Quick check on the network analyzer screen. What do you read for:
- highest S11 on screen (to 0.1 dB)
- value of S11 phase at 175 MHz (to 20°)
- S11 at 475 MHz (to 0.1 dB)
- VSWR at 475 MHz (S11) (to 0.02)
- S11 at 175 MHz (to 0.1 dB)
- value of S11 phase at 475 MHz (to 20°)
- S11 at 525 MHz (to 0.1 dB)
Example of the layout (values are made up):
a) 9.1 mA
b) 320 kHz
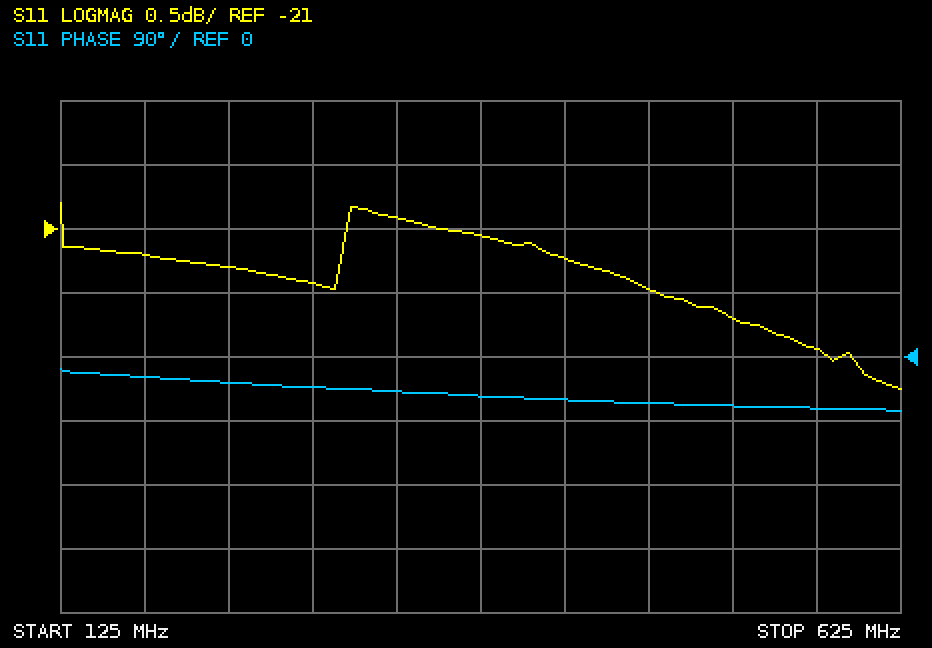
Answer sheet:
a) -20.8 dB
b) -20°
c) -21.5 dB
d) 1.18
e) -21.2 dB
f) -60°
g) -21.7 dB
